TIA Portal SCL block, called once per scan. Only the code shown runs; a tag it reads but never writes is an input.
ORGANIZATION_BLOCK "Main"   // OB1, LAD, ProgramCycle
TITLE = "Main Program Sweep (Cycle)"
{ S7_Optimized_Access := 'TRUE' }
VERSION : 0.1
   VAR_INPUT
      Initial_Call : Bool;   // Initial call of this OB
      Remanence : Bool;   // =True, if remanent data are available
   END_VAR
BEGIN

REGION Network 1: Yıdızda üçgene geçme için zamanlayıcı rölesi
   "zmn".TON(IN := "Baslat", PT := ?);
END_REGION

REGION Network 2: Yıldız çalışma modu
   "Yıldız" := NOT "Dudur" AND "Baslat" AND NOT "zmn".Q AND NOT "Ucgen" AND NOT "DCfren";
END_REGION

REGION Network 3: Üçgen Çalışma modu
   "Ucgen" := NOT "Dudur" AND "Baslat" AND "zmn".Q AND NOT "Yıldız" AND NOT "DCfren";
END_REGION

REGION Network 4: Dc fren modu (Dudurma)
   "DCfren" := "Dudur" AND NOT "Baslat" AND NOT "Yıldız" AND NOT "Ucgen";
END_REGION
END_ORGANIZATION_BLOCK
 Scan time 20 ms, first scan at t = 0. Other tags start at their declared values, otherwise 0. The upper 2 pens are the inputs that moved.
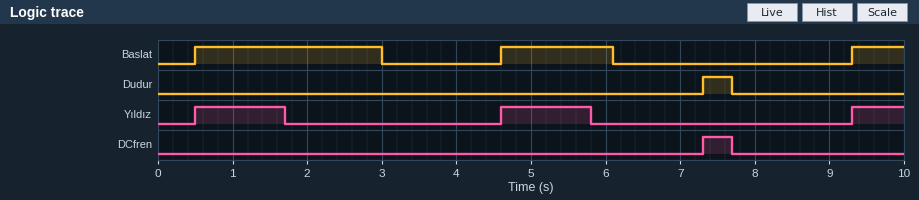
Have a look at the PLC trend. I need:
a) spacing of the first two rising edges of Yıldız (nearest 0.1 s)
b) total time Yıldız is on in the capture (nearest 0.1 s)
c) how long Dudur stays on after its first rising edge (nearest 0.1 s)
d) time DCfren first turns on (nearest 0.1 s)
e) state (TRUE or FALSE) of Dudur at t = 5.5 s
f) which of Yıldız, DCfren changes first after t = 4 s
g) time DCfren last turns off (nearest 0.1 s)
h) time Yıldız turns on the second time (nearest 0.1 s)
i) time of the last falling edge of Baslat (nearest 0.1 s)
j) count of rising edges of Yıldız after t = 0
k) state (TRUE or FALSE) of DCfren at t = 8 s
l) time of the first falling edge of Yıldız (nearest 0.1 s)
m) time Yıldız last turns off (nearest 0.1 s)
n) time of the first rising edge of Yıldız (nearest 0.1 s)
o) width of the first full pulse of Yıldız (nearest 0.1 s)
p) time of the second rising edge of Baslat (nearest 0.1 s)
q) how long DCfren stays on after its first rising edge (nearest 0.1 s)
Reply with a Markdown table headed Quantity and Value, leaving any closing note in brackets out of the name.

| Quantity | Value |
|---|---|
| spacing of the first two rising edges of Yıldız | 4.1 s |
| total time Yıldız is on in the capture | 3.1 s |
| how long Dudur stays on after its first rising edge | 0.4 s |
| time DCfren first turns on | 7.3 s |
| state (TRUE or FALSE) of Dudur at t = 5.5 s | FALSE |
| which of Yıldız, DCfren changes first after t = 4 s | Yıldız |
| time DCfren last turns off | 7.7 s |
| time Yıldız turns on the second time | 4.6 s |
| time of the last falling edge of Baslat | 6.1 s |
| count of rising edges of Yıldız after t = 0 | 3 |
| state (TRUE or FALSE) of DCfren at t = 8 s | FALSE |
| time of the first falling edge of Yıldız | 1.7 s |
| time Yıldız last turns off | 5.8 s |
| time of the first rising edge of Yıldız | 0.5 s |
| width of the first full pulse of Yıldız | 1.2 s |
| time of the second rising edge of Baslat | 4.6 s |
| how long DCfren stays on after its first rising edge | 0.4 s |
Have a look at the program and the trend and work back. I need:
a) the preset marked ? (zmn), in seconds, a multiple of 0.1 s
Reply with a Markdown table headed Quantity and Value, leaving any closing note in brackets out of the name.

| Quantity | Value |
|---|---|
| the preset marked ? (zmn), in seconds, a multiple of 0.1 s | 1.2 s |
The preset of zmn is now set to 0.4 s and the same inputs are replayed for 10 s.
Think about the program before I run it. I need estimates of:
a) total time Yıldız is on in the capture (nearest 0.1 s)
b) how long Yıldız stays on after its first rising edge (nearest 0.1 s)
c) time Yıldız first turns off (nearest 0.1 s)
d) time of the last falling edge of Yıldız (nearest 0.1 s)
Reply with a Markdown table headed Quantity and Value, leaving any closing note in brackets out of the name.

| Quantity | Value |
|---|---|
| total time Yıldız is on in the capture | 1.2 s |
| how long Yıldız stays on after its first rising edge | 0.4 s |
| time Yıldız first turns off | 0.9 s |
| time of the last falling edge of Yıldız | 9.7 s |
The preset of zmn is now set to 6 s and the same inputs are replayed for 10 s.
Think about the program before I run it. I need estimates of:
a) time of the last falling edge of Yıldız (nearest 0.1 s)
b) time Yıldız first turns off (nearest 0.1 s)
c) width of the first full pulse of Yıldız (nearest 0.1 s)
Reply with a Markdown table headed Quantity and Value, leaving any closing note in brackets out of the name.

| Quantity | Value |
|---|---|
| time of the last falling edge of Yıldız | 6.1 s |
| time Yıldız first turns off | 3.0 s |
| width of the first full pulse of Yıldız | 2.5 s |
